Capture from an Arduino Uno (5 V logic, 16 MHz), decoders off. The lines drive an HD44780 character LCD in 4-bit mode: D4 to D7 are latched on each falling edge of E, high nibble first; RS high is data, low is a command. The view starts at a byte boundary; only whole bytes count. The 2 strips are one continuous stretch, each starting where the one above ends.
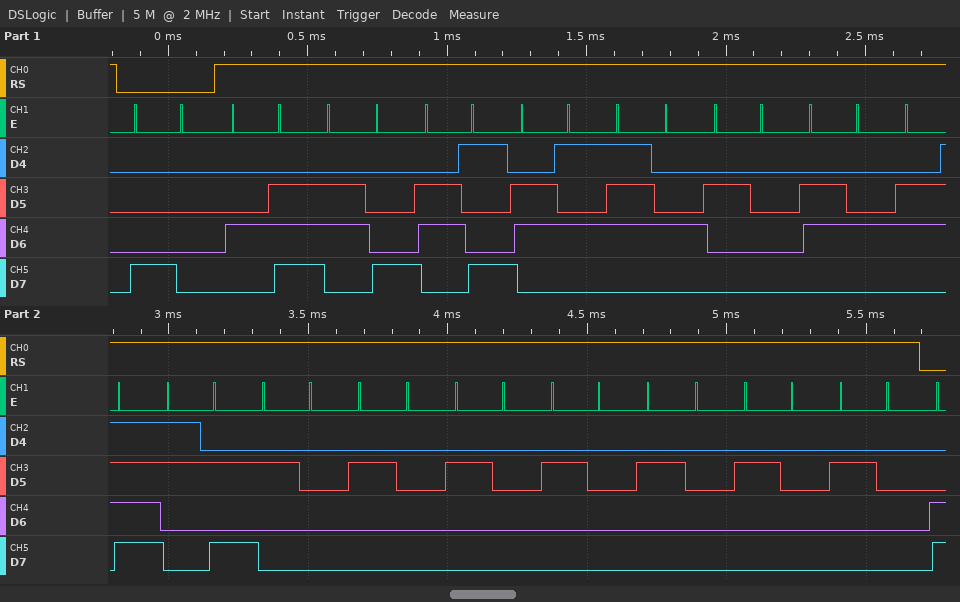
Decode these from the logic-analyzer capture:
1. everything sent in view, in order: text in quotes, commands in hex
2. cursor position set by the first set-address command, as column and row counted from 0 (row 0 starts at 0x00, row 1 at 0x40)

0x80 "Nhiet do:       "
column 0, row 0
